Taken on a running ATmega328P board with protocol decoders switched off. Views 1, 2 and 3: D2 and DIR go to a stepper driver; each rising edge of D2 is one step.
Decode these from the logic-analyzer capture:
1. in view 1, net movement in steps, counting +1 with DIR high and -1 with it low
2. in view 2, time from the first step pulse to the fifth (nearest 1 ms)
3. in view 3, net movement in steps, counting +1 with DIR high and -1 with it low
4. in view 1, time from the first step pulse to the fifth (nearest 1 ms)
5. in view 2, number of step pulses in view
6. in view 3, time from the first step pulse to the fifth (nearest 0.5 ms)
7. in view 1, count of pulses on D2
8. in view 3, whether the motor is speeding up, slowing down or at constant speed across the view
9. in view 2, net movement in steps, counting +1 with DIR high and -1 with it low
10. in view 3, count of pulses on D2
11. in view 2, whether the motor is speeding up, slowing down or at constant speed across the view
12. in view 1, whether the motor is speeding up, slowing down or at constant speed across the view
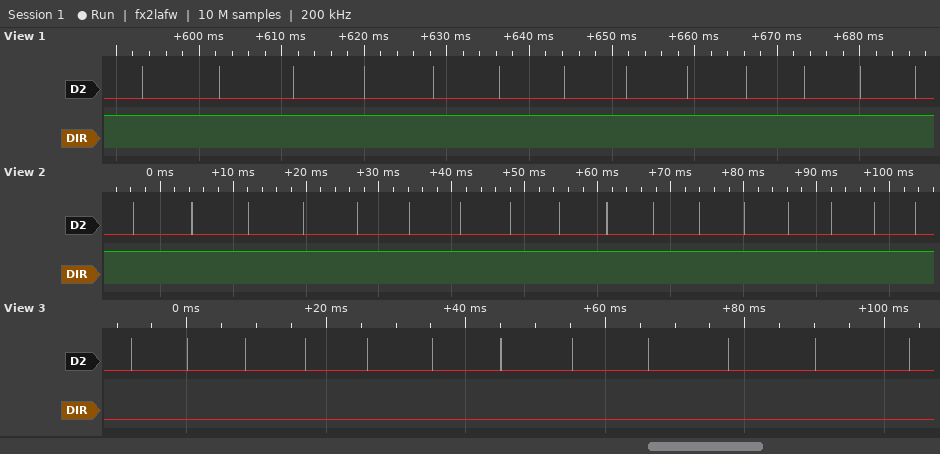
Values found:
+13
31 ms
-12
35 ms
17
34.0 ms
13
slowing down
+17
12
speeding up
speeding up
